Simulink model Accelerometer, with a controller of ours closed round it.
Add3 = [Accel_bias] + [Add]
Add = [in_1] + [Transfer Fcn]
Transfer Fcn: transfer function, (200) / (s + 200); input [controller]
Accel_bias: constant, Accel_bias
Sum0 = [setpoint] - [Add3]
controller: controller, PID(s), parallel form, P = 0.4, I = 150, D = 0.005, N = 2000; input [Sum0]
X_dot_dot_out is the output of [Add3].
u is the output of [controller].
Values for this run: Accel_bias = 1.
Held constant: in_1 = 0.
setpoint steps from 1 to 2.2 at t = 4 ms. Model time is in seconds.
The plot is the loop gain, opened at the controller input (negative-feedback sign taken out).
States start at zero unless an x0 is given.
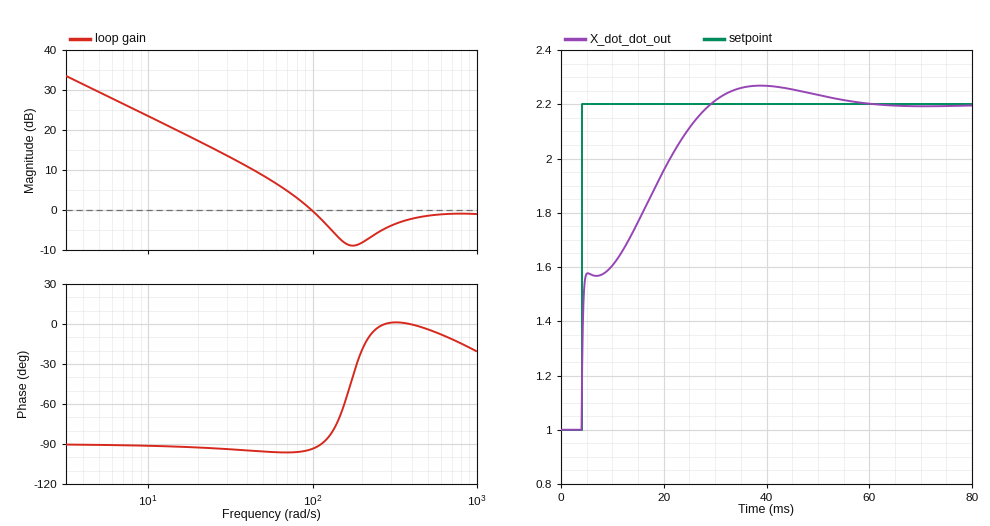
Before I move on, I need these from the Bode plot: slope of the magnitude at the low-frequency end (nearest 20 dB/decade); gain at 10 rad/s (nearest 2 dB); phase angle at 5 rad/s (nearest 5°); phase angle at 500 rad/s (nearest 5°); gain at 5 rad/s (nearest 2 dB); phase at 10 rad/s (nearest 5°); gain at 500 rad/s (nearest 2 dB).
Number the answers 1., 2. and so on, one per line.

1. -20 dB/decade
2. 24 dB
3. -90°
4. -5°
5. 30 dB
6. -90°
7. -2 dB
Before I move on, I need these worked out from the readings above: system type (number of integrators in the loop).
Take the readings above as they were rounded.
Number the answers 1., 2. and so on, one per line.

1. 1
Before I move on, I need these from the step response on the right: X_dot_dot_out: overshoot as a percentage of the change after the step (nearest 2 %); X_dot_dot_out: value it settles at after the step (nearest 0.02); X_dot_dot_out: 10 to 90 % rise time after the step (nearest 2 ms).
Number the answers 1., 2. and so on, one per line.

1. 6 %
2. 2.20
3. 20 ms
